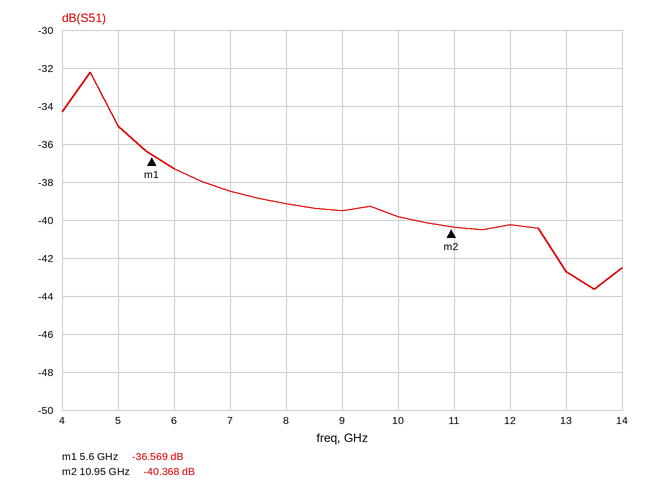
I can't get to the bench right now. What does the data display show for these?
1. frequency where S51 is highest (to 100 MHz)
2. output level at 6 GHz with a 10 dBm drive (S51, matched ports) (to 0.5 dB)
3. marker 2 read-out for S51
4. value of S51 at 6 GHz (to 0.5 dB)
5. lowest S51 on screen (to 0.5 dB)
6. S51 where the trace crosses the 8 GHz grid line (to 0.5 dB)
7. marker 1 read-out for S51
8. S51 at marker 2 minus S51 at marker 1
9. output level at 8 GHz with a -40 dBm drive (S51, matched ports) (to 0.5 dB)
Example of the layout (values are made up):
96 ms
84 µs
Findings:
4.5 GHz
-27.5 dBm
-40.368 dB
-37.5 dB
-43.5 dB
-39.0 dB
-36.569 dB
-3.799 dB
-79.0 dBm
